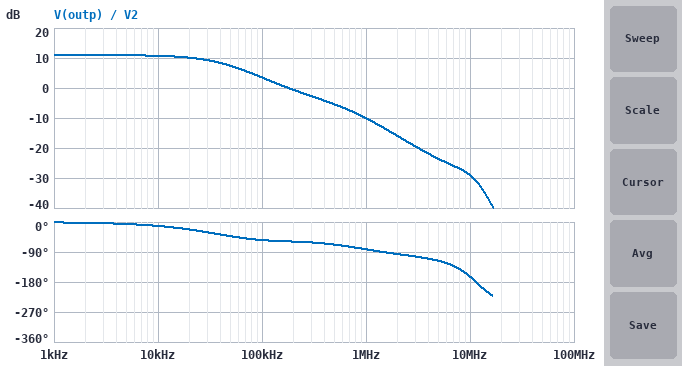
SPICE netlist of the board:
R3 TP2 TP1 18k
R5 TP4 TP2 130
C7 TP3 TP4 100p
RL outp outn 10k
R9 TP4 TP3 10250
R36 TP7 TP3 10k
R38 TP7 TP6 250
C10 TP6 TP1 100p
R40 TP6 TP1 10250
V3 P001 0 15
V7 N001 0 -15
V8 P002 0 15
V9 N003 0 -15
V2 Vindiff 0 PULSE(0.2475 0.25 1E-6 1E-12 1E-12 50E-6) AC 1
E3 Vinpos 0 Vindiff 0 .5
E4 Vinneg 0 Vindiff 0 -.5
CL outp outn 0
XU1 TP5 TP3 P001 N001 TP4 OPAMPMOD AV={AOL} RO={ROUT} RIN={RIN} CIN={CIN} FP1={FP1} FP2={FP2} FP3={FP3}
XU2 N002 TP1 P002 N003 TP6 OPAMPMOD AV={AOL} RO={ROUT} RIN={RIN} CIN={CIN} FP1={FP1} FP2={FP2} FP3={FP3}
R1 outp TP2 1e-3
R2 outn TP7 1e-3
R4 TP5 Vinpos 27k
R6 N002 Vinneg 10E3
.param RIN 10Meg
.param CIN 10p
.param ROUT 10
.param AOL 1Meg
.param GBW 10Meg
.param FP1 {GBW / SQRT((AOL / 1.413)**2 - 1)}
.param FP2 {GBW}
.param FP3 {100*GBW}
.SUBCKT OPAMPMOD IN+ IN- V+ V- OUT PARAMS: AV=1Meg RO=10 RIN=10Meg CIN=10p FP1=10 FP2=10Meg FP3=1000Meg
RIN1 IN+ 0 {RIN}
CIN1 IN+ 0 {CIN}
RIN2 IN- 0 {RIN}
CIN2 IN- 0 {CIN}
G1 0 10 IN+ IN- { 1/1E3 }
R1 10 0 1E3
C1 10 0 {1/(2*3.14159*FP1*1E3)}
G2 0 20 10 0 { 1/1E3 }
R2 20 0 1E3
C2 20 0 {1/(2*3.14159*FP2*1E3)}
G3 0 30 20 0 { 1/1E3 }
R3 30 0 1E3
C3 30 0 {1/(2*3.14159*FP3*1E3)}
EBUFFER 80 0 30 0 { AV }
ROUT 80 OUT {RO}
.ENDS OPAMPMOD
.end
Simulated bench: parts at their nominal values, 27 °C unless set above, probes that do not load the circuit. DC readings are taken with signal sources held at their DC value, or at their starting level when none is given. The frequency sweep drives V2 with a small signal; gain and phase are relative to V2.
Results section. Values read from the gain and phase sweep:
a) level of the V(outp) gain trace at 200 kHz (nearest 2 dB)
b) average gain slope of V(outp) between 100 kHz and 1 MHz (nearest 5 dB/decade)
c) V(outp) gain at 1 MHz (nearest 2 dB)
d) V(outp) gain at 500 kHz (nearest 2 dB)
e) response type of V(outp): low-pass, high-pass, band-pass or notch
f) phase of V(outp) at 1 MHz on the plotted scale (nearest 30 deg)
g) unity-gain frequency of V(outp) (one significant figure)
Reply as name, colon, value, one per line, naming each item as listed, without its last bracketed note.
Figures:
level of the V(outp) gain trace at 200 kHz: 0 dB
average gain slope of V(outp) between 100 kHz and 1 MHz: -15 dB/decade
V(outp) gain at 1 MHz: -10 dB
V(outp) gain at 500 kHz: -6 dB
response type of V(outp): low-pass, high-pass, band-pass or notch: low-pass
phase of V(outp) at 1 MHz on the plotted scale: -90 deg
unity-gain frequency of V(outp): 200 kHz
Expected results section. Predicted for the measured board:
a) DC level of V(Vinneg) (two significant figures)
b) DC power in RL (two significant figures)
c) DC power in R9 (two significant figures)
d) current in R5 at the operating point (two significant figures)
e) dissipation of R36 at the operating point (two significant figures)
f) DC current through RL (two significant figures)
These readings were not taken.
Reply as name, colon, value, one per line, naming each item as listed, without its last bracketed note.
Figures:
DC level of V(Vinneg): -120 mV
DC power in RL: 230 µW
DC power in R9: 59 µW
current in R5 at the operating point: 210 µA
dissipation of R36 at the operating point: 58 µW
DC current through RL: 150 µA
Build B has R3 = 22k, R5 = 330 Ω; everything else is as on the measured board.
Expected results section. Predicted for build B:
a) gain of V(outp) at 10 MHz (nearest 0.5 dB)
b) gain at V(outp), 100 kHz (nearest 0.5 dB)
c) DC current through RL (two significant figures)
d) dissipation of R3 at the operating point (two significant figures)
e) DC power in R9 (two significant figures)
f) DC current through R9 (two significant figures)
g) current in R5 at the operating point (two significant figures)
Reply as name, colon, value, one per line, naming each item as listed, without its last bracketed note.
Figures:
gain of V(outp) at 10 MHz: -30.0 dB
gain at V(outp), 100 kHz: 3.0 dB
DC current through RL: 110 µA
dissipation of R3 at the operating point: 28 µW
DC power in R9: 33 µW
DC current through R9: 57 µA
current in R5 at the operating point: 150 µA
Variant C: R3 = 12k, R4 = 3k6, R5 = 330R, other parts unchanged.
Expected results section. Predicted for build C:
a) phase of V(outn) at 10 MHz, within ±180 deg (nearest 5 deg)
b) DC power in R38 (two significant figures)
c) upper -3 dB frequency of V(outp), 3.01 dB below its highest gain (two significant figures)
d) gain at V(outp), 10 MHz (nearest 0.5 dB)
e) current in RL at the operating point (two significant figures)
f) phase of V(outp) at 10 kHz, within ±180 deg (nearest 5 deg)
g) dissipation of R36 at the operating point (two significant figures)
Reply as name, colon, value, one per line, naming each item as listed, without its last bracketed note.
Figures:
phase of V(outn) at 10 MHz, within ±180 deg: 20 deg
DC power in R38: 59 µW
upper -3 dB frequency of V(outp), 3.01 dB below its highest gain: 21 kHz
gain at V(outp), 10 MHz: -12.0 dB
current in RL at the operating point: 320 µA
phase of V(outp) at 10 kHz, within ±180 deg: -25 deg
dissipation of R36 at the operating point: 270 µW
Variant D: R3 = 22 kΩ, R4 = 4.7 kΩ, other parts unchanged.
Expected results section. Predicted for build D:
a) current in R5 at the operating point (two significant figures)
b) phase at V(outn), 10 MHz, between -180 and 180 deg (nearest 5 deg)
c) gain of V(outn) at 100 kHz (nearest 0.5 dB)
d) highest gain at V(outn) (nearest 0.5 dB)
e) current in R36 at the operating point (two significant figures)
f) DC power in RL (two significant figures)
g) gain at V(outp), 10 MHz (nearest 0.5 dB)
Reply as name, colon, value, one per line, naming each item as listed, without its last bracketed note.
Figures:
current in R5 at the operating point: 160 µA
phase at V(outn), 10 MHz, between -180 and 180 deg: 20 deg
gain of V(outn) at 100 kHz: -0.5 dB
highest gain at V(outn): 5.5 dB
current in R36 at the operating point: 59 µA
DC power in RL: 140 µW
gain at V(outp), 10 MHz: -13.5 dB
